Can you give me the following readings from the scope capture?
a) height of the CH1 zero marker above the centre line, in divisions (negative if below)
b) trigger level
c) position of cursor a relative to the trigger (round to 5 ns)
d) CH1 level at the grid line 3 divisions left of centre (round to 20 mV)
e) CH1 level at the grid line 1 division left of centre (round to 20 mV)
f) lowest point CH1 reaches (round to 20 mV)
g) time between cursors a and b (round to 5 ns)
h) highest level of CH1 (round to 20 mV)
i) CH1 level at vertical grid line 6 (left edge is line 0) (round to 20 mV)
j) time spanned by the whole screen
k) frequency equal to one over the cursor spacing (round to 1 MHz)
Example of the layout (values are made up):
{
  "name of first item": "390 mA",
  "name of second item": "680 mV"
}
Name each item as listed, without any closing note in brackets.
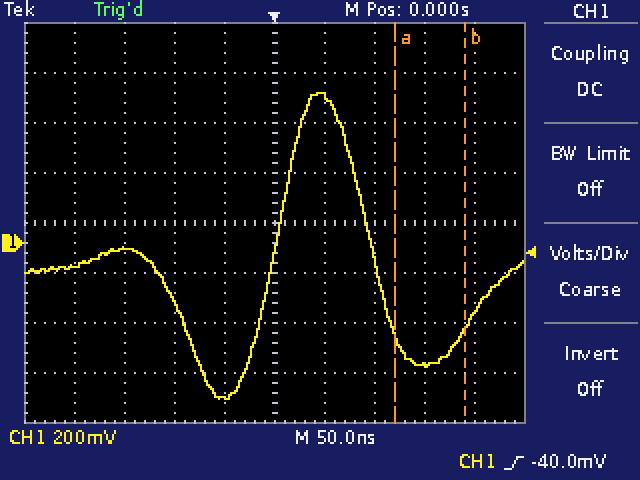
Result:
{
  "height of the CH1 zero marker above the centre line, in divisions": "-0.4 div",
  "trigger level": "-40.0 mV",
  "position of cursor a relative to the trigger": "+120 ns",
  "CH1 level at the grid line 3 divisions left of centre": "-20 mV",
  "CH1 level at the grid line 1 division left of centre": "-620 mV",
  "lowest point CH1 reaches": "-620 mV",
  "time between cursors a and b": "70 ns",
  "highest level of CH1": "600 mV",
  "CH1 level at vertical grid line 6 (left edge is line 0)": "580 mV",
  "time spanned by the whole screen": "500 ns",
  "frequency equal to one over the cursor spacing": "14 MHz"
}
